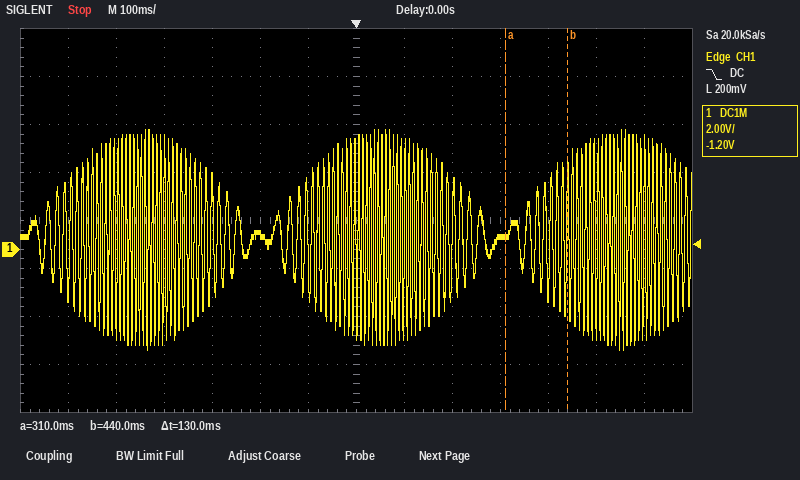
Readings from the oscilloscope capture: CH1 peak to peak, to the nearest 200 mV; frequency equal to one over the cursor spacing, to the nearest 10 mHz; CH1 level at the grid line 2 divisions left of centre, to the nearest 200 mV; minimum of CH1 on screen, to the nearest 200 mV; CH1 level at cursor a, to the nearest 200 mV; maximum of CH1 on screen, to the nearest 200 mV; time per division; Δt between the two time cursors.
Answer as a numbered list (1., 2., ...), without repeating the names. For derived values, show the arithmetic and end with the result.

1. 5.0 V − (-4.2 V) = 9.2 V
2. 1 / 130 ms ≈ 7.69 Hz
3. 600 mV
4. -4.2 V
5. 600 mV
6. 5.0 V
7. 100 ms
8. 130 ms
